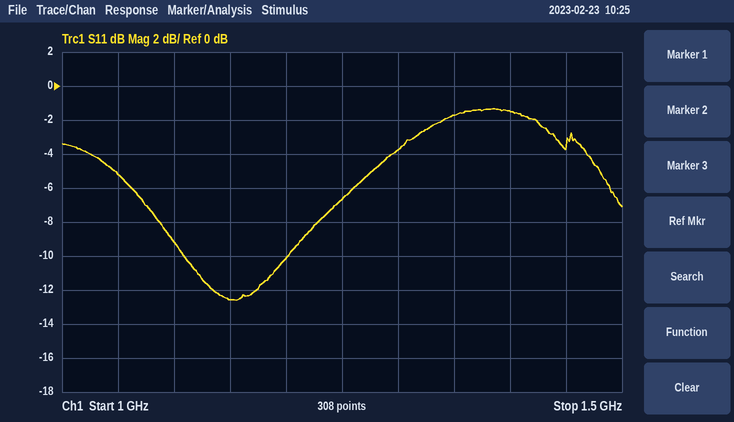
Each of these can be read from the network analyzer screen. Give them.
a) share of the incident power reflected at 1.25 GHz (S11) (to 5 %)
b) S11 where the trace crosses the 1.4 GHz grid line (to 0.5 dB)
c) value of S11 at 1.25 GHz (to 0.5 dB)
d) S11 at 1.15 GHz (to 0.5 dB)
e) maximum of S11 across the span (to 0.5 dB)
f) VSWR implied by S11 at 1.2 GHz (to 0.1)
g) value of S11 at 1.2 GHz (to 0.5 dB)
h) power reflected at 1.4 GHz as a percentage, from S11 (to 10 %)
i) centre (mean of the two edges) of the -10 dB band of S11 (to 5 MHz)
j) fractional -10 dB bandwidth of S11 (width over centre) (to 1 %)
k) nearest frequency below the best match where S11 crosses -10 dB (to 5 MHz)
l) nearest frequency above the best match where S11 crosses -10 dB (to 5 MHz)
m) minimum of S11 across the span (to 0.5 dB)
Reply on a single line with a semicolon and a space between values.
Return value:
20 %; -1.5 dB; -6.5 dB; -12.5 dB; -1.5 dB; 1.9; -10.0 dB; 70 %; 1.155 GHz; 8 %; 1.110 GHz; 1.200 GHz; -12.5 dB
